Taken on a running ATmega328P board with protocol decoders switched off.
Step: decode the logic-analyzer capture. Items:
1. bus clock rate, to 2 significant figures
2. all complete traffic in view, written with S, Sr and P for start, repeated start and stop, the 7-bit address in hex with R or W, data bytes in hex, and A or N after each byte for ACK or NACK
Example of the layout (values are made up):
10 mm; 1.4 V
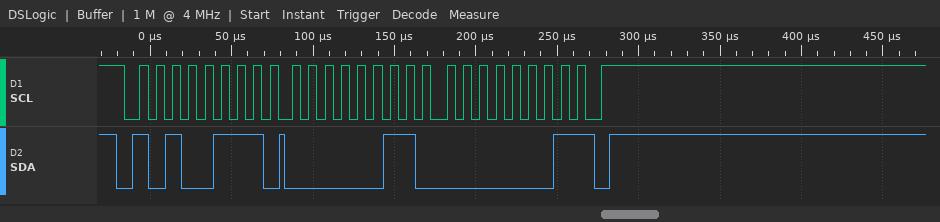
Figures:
100 kHz; S 53R A 03 A 01 N P
